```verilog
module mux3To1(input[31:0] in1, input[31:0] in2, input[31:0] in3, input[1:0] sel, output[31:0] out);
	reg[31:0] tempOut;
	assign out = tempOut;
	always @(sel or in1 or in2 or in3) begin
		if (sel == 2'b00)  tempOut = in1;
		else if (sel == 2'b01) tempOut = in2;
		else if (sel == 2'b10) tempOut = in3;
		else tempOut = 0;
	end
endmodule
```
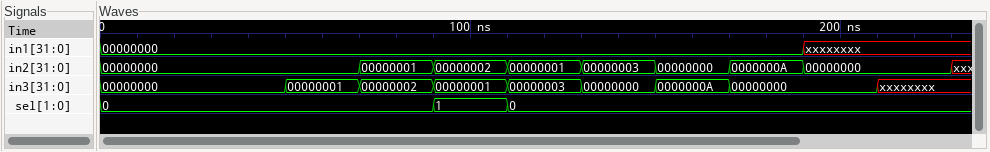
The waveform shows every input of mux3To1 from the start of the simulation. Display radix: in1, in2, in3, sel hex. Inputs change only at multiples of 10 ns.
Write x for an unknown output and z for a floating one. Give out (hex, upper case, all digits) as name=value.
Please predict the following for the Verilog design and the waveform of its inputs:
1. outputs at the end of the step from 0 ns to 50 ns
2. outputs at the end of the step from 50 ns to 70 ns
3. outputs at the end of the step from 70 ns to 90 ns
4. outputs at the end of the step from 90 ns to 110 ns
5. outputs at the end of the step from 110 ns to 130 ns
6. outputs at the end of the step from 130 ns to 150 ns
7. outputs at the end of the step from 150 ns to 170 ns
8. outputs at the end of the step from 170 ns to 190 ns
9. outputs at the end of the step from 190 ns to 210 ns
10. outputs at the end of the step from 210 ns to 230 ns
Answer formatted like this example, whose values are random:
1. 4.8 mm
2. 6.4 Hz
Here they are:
1. out=00000000
2. out=00000000
3. out=00000000
4. out=00000002
5. out=00000000
6. out=00000000
7. out=00000000
8. out=00000000
9. out=x
10. out=x
